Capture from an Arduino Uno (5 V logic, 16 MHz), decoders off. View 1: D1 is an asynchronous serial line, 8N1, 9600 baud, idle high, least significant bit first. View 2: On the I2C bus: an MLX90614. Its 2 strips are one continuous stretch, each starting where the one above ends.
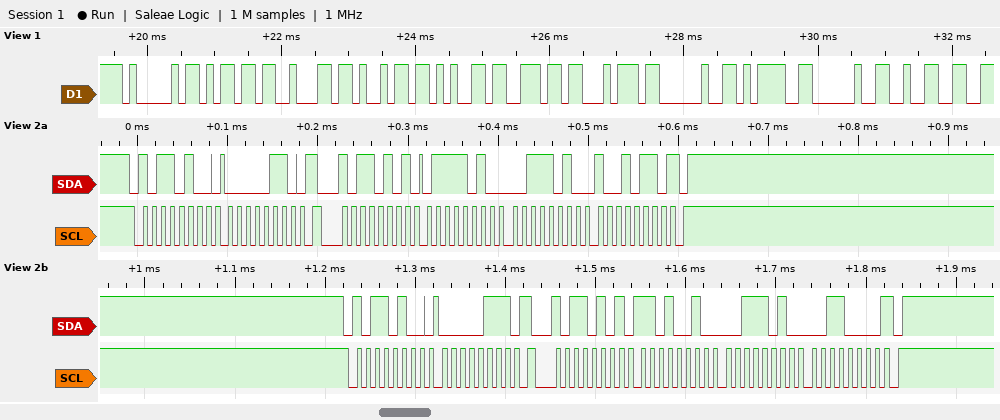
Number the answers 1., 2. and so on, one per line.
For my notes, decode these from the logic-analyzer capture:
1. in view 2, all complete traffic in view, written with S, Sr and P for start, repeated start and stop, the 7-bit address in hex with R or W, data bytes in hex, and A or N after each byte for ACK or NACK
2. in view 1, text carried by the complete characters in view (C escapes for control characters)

1. S 5AW A 06 A Sr 5AR A 7A A 3A A 96 N P S 5AW A 07 A Sr 5AR A D2 A 3A A 30 N P
2. "Ambient = 2"
